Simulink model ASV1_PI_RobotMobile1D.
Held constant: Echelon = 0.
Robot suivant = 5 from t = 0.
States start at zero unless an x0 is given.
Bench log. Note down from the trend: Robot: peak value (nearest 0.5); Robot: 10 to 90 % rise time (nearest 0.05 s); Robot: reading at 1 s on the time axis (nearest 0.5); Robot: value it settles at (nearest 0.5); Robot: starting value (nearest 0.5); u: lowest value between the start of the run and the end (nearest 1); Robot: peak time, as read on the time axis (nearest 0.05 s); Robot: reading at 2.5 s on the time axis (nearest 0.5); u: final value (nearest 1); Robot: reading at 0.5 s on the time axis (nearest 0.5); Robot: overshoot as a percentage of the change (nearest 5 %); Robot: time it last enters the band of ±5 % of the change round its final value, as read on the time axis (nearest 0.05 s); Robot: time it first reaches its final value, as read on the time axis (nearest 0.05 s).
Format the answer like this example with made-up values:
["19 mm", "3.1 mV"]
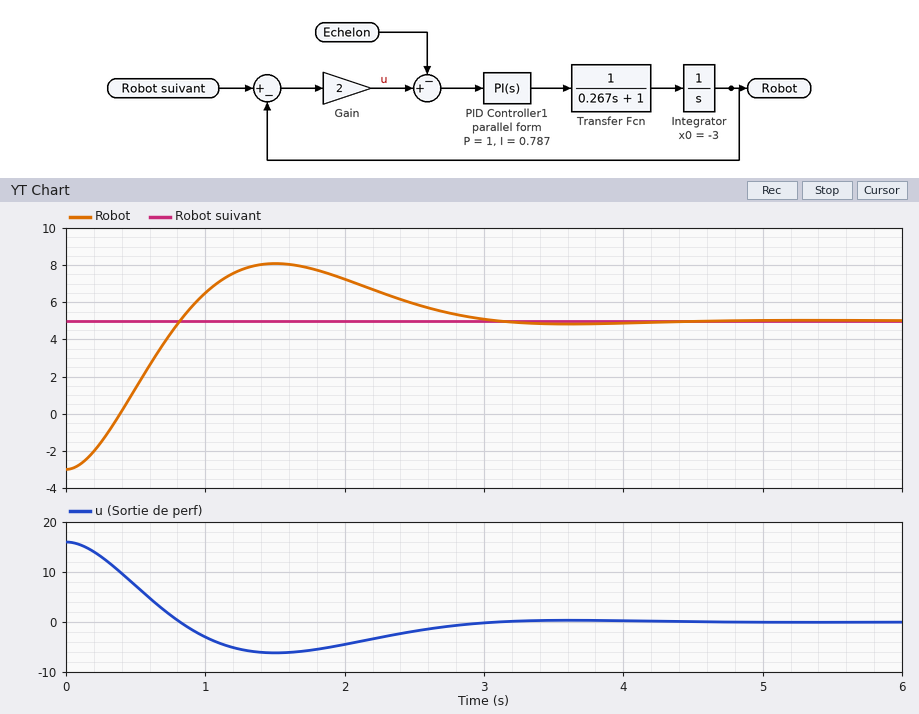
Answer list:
["8.0", "0.55 s", "6.5", "5.0", "-3.0", "-6", "1.50 s", "6.0", "0", "1.5", "40 %", "2.75 s", "0.80 s"]
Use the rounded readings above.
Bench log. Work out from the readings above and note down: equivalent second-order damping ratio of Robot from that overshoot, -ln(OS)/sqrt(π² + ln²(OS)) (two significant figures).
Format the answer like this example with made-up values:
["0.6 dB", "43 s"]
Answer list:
["0.28"]
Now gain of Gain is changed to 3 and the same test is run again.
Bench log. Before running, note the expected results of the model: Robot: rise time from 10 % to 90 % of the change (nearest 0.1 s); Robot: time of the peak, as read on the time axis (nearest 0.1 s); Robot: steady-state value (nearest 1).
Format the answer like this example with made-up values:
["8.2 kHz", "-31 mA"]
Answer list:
["0.4 s", "1.1 s", "5"]
